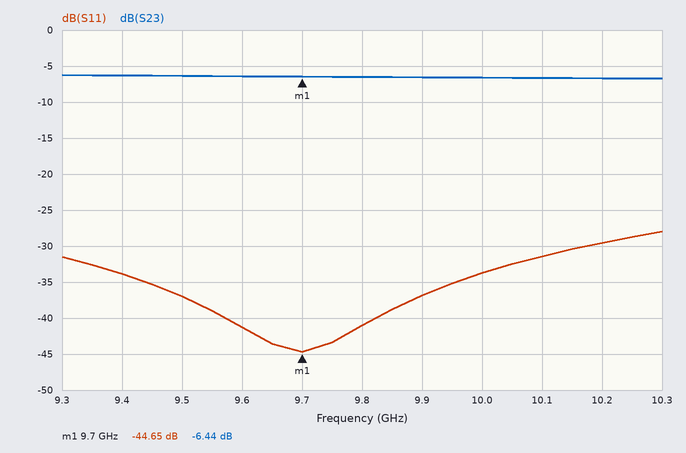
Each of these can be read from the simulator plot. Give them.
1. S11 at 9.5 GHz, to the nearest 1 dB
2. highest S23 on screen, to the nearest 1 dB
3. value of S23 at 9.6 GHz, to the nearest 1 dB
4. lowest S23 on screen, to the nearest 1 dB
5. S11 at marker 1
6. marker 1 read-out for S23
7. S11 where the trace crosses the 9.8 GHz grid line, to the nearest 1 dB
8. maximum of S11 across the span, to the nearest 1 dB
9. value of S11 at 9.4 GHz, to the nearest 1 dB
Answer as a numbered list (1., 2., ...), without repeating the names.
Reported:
1. -37 dB
2. -6 dB
3. -6 dB
4. -7 dB
5. -44.65 dB
6. -6.44 dB
7. -41 dB
8. -28 dB
9. -34 dB
